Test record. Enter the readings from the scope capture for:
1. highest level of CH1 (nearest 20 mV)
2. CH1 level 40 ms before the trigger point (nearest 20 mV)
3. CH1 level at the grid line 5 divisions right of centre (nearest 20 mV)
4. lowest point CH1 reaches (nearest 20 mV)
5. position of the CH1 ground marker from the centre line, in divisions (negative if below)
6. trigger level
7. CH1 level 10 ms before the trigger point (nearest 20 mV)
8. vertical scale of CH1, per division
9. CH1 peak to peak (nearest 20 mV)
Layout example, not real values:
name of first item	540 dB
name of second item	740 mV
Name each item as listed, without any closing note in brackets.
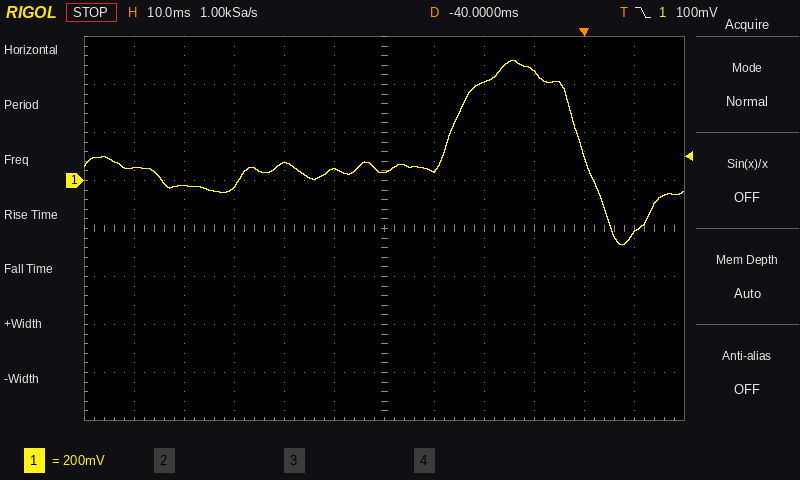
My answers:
highest level of CH1	500 mV
CH1 level 40 ms before the trigger point	40 mV
CH1 level at the grid line 5 divisions right of centre	-220 mV
lowest point CH1 reaches	-260 mV
position of the CH1 ground marker from the centre line, in divisions	+1.0 div
trigger level	100 mV
CH1 level 10 ms before the trigger point	460 mV
vertical scale of CH1, per division	200 mV
CH1 peak to peak	760 mV
